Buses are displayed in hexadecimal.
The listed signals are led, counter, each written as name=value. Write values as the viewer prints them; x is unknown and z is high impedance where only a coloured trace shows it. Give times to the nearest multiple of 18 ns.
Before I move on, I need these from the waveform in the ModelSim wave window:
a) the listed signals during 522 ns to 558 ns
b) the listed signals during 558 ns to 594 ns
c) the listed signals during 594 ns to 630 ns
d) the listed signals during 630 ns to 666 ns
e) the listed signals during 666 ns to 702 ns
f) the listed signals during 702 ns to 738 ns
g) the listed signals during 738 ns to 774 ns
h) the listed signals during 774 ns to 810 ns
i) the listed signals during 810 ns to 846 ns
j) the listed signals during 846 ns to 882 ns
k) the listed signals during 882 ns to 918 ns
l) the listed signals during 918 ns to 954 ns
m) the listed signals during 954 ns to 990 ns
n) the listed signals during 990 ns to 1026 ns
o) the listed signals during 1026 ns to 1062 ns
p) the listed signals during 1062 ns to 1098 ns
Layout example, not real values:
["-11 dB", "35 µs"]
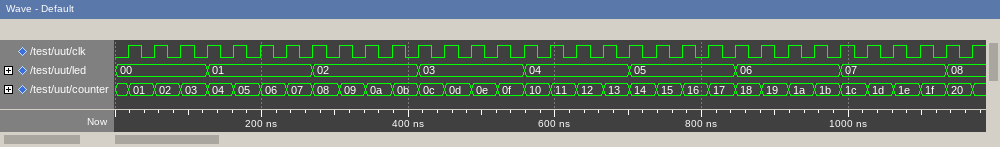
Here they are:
["led=03, counter=0f", "led=04, counter=10", "led=04, counter=11", "led=04, counter=12", "led=04, counter=13", "led=05, counter=14", "led=05, counter=15", "led=05, counter=16", "led=05, counter=17", "led=06, counter=18", "led=06, counter=19", "led=06, counter=1a", "led=06, counter=1b", "led=07, counter=1c", "led=07, counter=1d", "led=07, counter=1e"]
